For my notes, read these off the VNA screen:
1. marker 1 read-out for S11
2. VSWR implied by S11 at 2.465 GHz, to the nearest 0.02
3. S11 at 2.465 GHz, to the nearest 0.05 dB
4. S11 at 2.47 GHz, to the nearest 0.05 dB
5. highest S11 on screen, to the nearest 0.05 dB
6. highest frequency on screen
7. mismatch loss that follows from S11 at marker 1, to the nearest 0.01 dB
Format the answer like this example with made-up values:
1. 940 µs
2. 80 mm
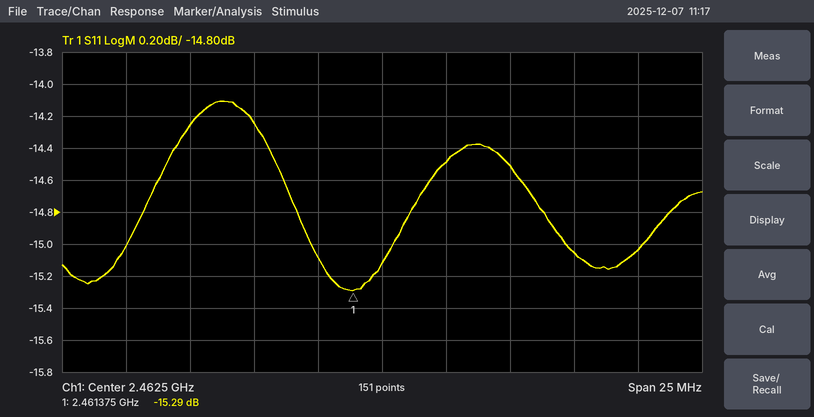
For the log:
1. -15.29 dB
2. 1.46
3. -14.50 dB
4. -15.05 dB
5. -14.10 dB
6. 2.475 GHz
7. 0.13 dB
